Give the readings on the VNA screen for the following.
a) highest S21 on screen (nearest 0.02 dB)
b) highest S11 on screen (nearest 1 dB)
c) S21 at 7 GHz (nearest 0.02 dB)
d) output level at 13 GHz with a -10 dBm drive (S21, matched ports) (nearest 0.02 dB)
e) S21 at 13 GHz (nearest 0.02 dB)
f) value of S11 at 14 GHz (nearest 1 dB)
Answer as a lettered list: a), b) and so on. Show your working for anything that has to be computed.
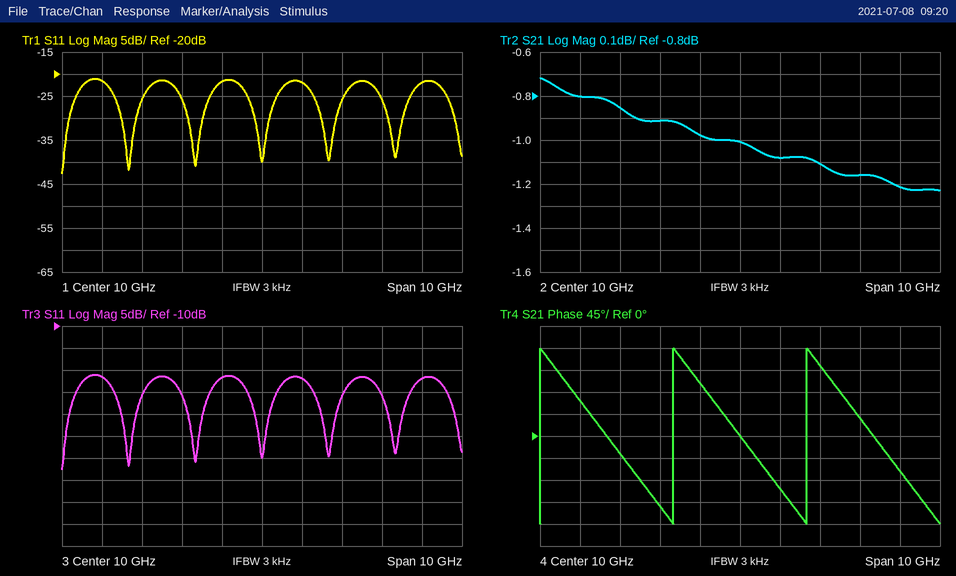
a) -0.72 dB
b) -21 dB
c) -0.86 dB
d) -10 dBm + (-1.16 dB) = -11.16 dBm
e) -1.16 dB
f) -22 dB
